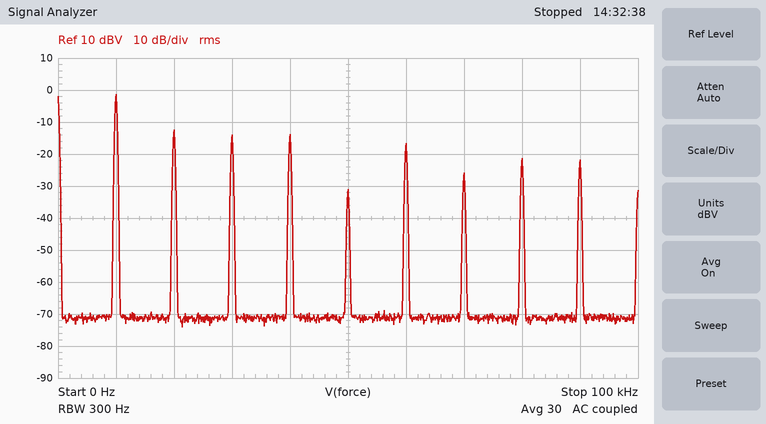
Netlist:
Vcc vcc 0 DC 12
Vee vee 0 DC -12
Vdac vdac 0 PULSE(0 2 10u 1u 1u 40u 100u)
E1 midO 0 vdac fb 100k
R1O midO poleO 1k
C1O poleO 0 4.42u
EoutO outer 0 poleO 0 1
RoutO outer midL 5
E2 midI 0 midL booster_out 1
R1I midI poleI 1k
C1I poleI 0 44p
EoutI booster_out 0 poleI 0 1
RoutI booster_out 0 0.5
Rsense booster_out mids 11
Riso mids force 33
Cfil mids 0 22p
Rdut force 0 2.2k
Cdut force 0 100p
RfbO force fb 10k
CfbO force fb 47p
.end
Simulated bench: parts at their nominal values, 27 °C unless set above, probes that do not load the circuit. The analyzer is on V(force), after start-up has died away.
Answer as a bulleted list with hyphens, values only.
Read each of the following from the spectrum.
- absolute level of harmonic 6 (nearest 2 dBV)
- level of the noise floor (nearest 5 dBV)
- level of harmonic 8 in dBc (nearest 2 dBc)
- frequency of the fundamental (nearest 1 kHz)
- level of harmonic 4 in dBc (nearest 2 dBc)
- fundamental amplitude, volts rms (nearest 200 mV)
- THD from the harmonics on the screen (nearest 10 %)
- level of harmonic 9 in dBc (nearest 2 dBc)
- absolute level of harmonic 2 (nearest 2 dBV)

- -16 dBV
- -70 dBV
- -20 dBc
- 10 kHz
- -12 dBc
- 800 mV
- 50 %
- -20 dBc
- -12 dBV
